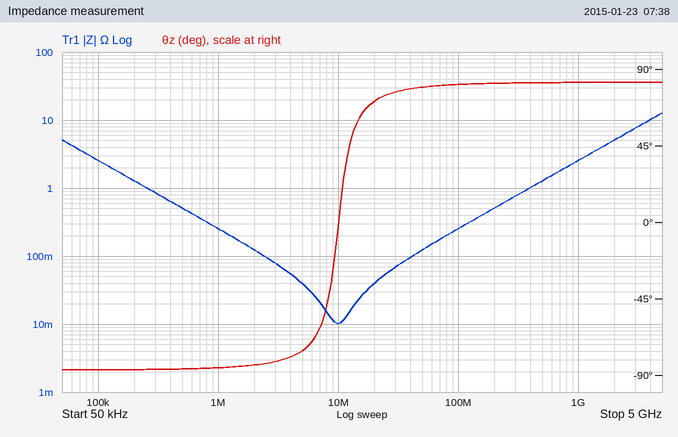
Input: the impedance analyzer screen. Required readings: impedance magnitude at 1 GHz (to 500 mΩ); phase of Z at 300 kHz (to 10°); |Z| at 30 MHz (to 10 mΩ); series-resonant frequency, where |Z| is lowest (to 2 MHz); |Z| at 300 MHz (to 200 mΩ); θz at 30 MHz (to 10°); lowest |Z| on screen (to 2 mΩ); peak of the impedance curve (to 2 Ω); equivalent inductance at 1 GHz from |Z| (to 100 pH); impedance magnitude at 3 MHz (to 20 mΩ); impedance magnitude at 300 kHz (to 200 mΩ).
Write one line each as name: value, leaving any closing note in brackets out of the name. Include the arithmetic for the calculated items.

impedance magnitude at 1 GHz: 2.5 Ω
phase of Z at 300 kHz: -90°
|Z| at 30 MHz: 70 mΩ
series-resonant frequency, where |Z| is lowest: 10 MHz
|Z| at 300 MHz: 800 mΩ
θz at 30 MHz: 80°
lowest |Z| on screen: 10 mΩ
peak of the impedance curve: 12 Ω
equivalent inductance at 1 GHz from |Z|: L = 2.5 Ω/(2π × 1 GHz) ≈ 398 pH, so 400 pH to the nearest 100 pH
impedance magnitude at 3 MHz: 80 mΩ
impedance magnitude at 300 kHz: 800 mΩ
